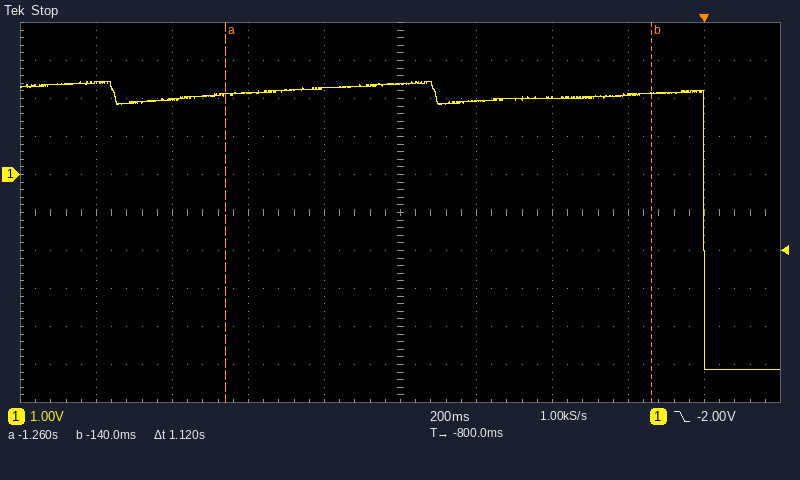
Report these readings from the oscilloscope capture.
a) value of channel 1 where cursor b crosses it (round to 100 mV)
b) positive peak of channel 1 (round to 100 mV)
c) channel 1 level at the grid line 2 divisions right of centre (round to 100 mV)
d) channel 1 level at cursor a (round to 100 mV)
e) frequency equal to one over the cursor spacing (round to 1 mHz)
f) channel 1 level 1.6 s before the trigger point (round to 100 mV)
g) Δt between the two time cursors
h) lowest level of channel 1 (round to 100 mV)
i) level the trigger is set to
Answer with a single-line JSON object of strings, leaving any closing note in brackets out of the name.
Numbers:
{"value of channel 1 where cursor b crosses it": "2.1 V", "positive peak of channel 1": "2.4 V", "channel 1 level at the grid line 2 divisions right of centre": "2.0 V", "channel 1 level at cursor a": "2.1 V", "frequency equal to one over the cursor spacing": "893 mHz", "channel 1 level 1.6 s before the trigger point": "2.4 V", "Δt between the two time cursors": "1.12 s", "lowest level of channel 1": "-5.1 V", "level the trigger is set to": "-2.00 V"}
